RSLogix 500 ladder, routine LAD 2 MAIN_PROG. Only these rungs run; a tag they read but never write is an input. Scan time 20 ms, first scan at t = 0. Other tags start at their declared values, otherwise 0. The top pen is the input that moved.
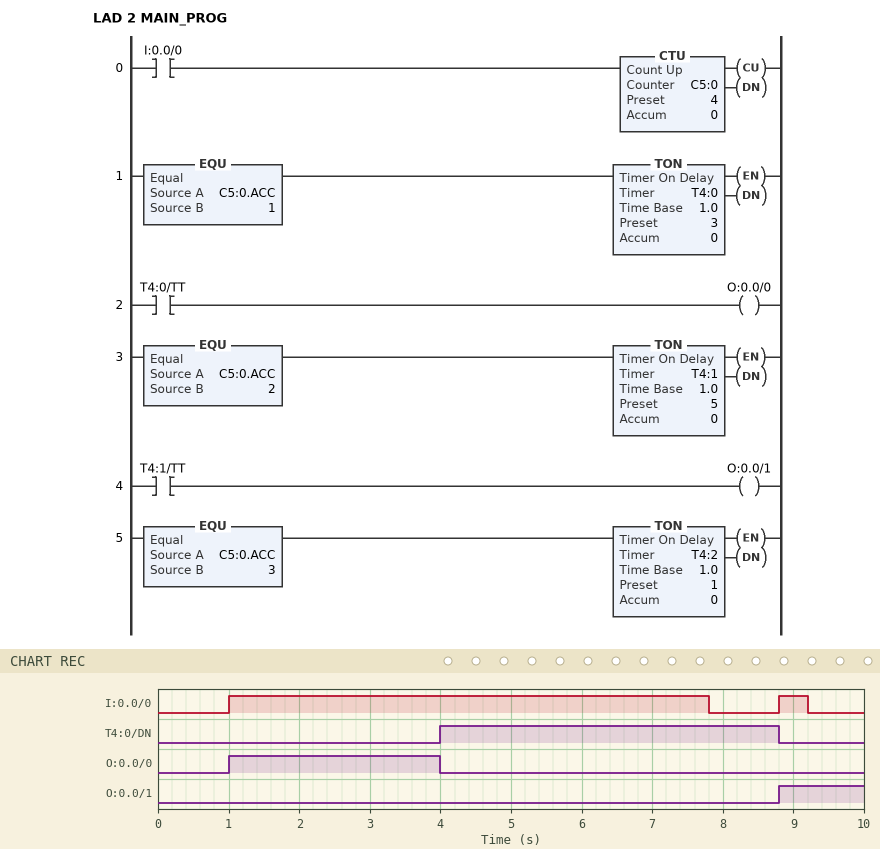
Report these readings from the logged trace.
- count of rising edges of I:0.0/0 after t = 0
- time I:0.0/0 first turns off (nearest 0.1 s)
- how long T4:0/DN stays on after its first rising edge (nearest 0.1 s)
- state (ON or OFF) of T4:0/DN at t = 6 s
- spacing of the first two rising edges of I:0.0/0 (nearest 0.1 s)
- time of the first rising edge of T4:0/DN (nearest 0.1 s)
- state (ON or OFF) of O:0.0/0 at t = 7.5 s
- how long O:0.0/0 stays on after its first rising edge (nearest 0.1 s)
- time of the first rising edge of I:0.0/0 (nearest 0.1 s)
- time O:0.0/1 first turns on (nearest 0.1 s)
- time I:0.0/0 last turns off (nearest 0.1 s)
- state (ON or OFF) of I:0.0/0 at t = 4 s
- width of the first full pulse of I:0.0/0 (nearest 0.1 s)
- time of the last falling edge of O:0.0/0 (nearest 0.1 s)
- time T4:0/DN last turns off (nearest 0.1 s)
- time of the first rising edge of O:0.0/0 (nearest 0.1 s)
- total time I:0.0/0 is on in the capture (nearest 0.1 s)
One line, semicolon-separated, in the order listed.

2; 7.8 s; 4.8 s; ON; 7.8 s; 4.0 s; OFF; 3.0 s; 1.0 s; 8.8 s; 9.2 s; ON; 6.8 s; 4.0 s; 8.8 s; 1.0 s; 7.2 s
